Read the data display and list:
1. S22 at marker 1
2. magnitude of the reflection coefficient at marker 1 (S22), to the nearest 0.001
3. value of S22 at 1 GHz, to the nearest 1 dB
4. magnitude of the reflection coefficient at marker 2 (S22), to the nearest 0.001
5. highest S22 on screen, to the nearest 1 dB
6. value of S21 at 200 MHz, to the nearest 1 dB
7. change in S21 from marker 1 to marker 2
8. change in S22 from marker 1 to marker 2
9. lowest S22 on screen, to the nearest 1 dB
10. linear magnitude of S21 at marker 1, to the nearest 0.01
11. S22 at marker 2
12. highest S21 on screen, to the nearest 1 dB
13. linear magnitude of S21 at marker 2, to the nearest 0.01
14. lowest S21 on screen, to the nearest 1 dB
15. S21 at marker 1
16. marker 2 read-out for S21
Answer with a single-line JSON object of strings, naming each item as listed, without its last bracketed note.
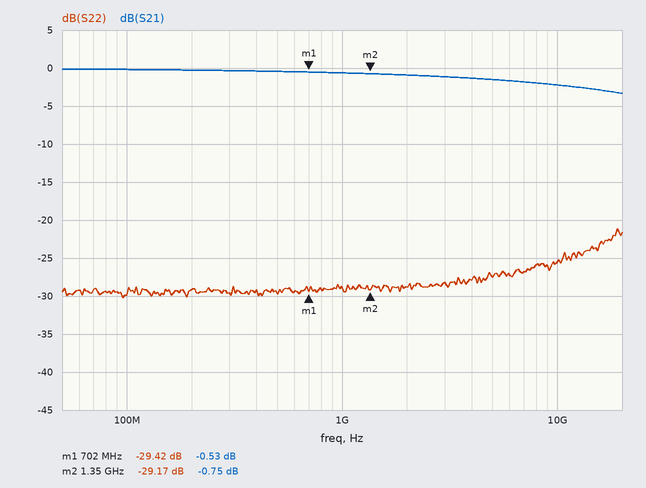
{"S22 at marker 1": "-29.42 dB", "magnitude of the reflection coefficient at marker 1 (S22), to the nearest 0.001": "0.034", "value of S22 at 1 GHz, to the nearest 1 dB": "-29 dB", "magnitude of the reflection coefficient at marker 2 (S22), to the nearest 0.001": "0.035", "highest S22 on screen, to the nearest 1 dB": "-21 dB", "value of S21 at 200 MHz, to the nearest 1 dB": "0 dB", "change in S21 from marker 1 to marker 2": "-0.22 dB", "change in S22 from marker 1 to marker 2": "0.25 dB", "lowest S22 on screen, to the nearest 1 dB": "-30 dB", "linear magnitude of S21 at marker 1, to the nearest 0.01": "0.94", "S22 at marker 2": "-29.17 dB", "highest S21 on screen, to the nearest 1 dB": "0 dB", "linear magnitude of S21 at marker 2, to the nearest 0.01": "0.92", "lowest S21 on screen, to the nearest 1 dB": "-3 dB", "S21 at marker 1": "-0.53 dB", "marker 2 read-out for S21": "-0.75 dB"}
